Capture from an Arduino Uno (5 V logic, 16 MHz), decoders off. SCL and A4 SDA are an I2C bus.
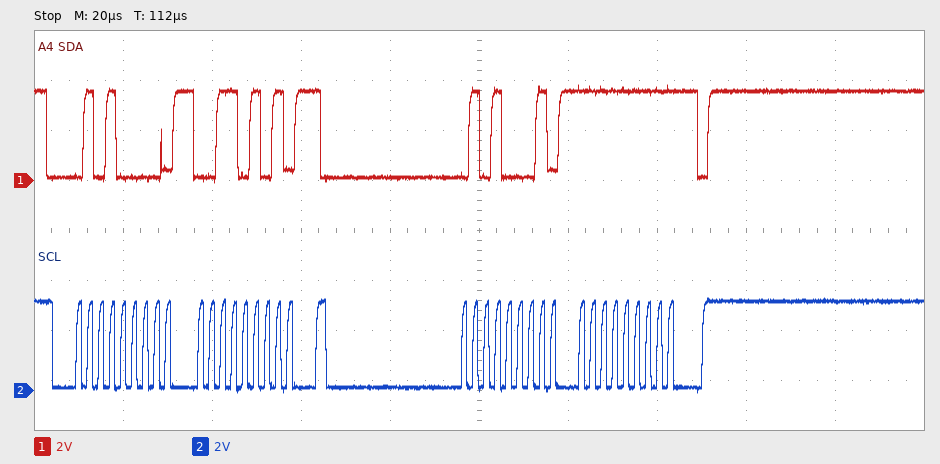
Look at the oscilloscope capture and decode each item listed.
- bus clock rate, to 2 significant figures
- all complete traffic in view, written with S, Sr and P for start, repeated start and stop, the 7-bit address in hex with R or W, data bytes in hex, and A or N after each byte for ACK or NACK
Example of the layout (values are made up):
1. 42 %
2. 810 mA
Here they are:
1. 400 kHz
2. S 28W A 35 A Sr 28R A FF N P
